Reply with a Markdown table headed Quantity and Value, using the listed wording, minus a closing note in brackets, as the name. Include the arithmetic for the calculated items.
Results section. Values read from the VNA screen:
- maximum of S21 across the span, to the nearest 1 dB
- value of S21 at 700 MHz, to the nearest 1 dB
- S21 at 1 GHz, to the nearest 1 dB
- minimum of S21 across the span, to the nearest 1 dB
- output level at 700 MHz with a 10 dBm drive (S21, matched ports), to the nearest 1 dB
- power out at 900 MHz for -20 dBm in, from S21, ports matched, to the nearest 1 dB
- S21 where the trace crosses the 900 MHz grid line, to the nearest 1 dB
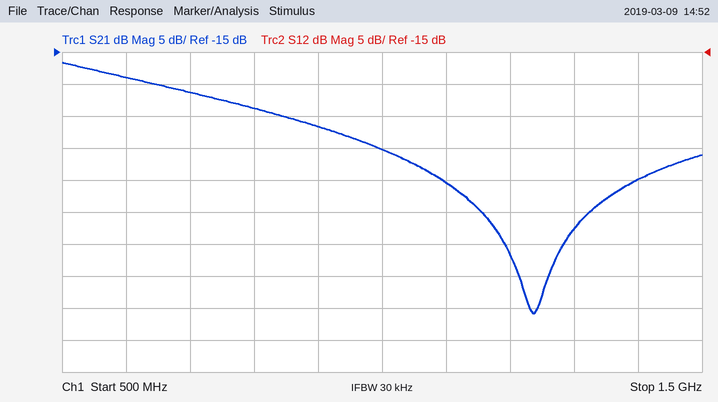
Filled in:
| Quantity | Value |
|---|---|
| maximum of S21 across the span, to the nearest 1 dB | -17 dB |
| value of S21 at 700 MHz, to the nearest 1 dB | -21 dB |
| S21 at 1 GHz, to the nearest 1 dB | -30 dB |
| minimum of S21 across the span, to the nearest 1 dB | -56 dB |
| output level at 700 MHz with a 10 dBm drive (S21, matched ports), to the nearest 1 dB | 10 dBm + (-21 dB) = -11 dBm |
| power out at 900 MHz for -20 dBm in, from S21, ports matched, to the nearest 1 dB | -20 dBm + (-27 dB) = -47 dBm |
| S21 where the trace crosses the 900 MHz grid line, to the nearest 1 dB | -27 dB |
